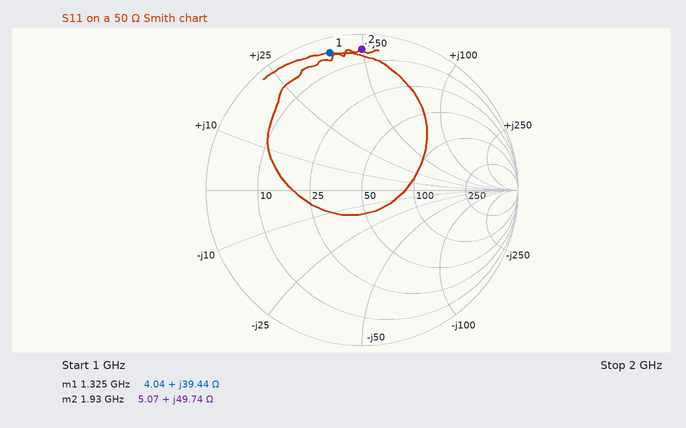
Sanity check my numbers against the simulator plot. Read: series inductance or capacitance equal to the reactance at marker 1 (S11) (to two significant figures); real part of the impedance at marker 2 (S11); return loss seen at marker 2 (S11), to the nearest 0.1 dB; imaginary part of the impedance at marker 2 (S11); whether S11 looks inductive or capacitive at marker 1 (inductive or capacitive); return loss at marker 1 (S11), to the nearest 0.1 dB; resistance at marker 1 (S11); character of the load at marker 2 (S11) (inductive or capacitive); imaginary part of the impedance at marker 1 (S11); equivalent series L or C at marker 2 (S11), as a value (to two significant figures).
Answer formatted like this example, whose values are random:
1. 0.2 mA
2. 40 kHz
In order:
1. 4.7 nH
2. 5.07 Ω
3. 0.9 dB
4. +49.74 Ω
5. inductive
6. 0.9 dB
7. 4.04 Ω
8. inductive
9. +39.44 Ω
10. 4.1 nH
